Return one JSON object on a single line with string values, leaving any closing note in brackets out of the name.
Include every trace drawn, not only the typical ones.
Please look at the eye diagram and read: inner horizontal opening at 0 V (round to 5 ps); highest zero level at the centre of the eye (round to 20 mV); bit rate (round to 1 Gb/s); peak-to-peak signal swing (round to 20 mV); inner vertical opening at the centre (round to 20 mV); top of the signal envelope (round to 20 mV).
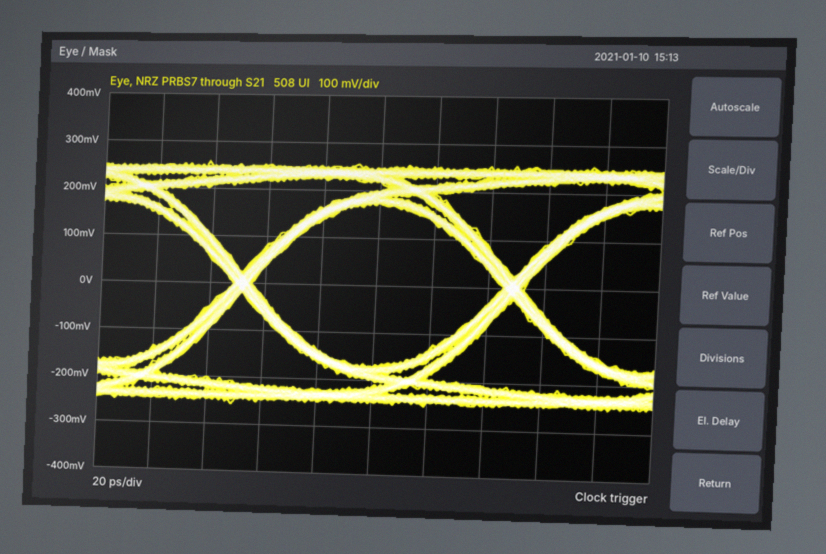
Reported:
{"inner horizontal opening at 0 V": "90 ps", "highest zero level at the centre of the eye": "-180 mV", "bit rate": "10 Gb/s", "peak-to-peak signal swing": "520 mV", "inner vertical opening at the centre": "340 mV", "top of the signal envelope": "260 mV"}
